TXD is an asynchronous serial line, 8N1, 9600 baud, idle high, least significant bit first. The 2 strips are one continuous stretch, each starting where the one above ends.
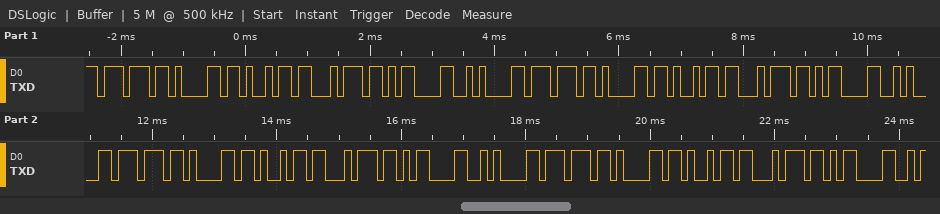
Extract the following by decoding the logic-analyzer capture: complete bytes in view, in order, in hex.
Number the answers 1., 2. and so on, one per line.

1. 77 61 69 74 0D 0A 77 61 69 74 0D 0A 77 61 69 74 0D 0A 77 61 69 74 0D
